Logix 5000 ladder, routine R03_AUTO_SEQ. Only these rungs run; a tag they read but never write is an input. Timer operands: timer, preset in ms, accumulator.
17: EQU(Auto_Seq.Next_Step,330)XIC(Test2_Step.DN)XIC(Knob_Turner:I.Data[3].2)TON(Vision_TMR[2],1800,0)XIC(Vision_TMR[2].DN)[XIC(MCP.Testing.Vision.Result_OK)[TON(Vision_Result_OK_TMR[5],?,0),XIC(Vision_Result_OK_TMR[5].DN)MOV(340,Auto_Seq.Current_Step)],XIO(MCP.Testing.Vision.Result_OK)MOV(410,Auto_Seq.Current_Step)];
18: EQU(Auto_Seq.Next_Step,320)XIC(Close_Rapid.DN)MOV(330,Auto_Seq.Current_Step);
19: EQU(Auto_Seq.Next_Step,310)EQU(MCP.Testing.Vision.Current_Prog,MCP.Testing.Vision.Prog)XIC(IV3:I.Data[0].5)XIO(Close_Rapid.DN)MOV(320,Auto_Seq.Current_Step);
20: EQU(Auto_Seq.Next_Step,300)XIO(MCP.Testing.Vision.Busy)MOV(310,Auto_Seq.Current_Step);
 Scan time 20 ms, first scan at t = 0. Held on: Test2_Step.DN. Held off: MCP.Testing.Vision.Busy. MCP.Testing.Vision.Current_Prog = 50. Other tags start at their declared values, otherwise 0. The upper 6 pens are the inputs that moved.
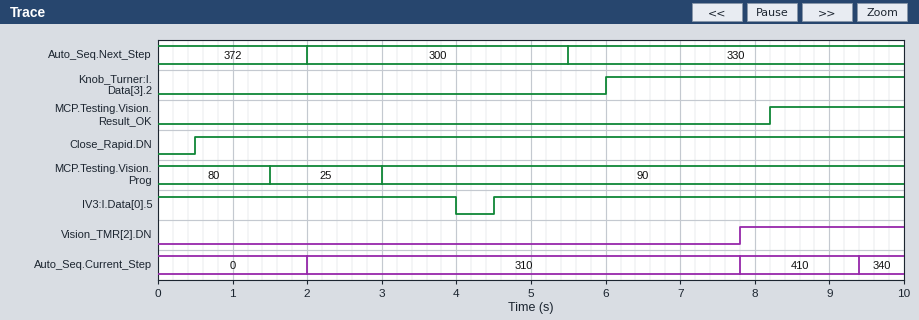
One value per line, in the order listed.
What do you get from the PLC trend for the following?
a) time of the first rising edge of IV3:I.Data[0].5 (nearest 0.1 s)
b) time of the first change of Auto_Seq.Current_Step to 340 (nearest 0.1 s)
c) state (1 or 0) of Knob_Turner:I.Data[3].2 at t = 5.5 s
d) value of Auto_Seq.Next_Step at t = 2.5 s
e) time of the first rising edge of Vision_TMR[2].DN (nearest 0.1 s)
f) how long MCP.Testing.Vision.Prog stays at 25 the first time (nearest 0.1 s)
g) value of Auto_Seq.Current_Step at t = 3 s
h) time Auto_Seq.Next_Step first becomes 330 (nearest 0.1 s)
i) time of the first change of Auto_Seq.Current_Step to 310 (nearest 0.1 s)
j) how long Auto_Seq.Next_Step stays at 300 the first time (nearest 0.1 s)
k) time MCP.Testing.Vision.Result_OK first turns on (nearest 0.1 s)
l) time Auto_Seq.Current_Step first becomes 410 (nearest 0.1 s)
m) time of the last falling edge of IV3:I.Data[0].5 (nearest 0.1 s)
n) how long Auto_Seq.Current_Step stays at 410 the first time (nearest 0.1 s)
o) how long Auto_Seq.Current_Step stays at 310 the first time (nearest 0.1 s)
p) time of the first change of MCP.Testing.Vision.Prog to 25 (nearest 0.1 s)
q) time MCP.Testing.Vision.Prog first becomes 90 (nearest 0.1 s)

4.5 s
9.4 s
0
300
7.8 s
1.5 s
310
5.5 s
2.0 s
3.5 s
8.2 s
7.8 s
4.0 s
1.6 s
5.8 s
1.5 s
3.0 s
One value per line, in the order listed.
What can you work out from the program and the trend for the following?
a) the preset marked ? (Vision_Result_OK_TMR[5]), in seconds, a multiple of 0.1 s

1.2 s
